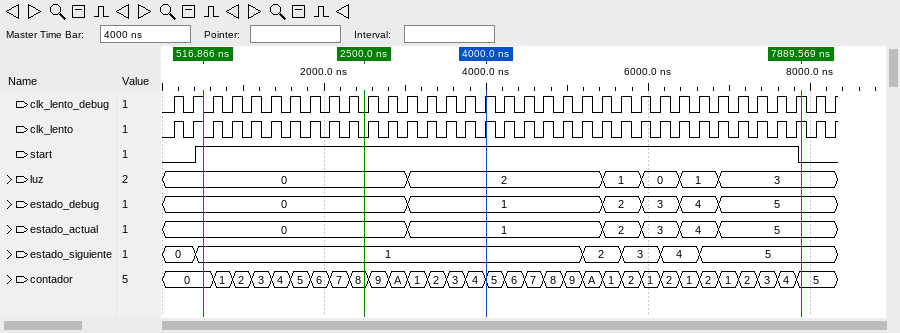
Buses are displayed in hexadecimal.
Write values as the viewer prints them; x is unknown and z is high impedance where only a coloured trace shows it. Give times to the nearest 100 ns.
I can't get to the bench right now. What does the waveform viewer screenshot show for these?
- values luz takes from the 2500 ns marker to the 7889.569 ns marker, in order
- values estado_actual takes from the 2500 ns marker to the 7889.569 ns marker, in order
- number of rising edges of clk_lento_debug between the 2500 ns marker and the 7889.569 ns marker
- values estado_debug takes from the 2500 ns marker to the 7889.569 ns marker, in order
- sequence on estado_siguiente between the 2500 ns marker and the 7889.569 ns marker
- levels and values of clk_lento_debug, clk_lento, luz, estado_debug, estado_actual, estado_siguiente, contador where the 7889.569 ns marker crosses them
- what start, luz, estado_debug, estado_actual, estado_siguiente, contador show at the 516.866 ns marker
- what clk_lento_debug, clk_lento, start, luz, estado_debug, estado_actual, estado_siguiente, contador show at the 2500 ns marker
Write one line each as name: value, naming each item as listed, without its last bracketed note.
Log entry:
values luz takes from the 2500 ns marker to the 7889.569 ns marker, in order: 0, 2, 1, 0, 1, 3
values estado_actual takes from the 2500 ns marker to the 7889.569 ns marker, in order: 0, 1, 2, 3, 4, 5
number of rising edges of clk_lento_debug between the 2500 ns marker and the 7889.569 ns marker: 23
values estado_debug takes from the 2500 ns marker to the 7889.569 ns marker, in order: 0, 1, 2, 3, 4, 5
sequence on estado_siguiente between the 2500 ns marker and the 7889.569 ns marker: 1, 2, 3, 4, 5
levels and values of clk_lento_debug, clk_lento, luz, estado_debug, estado_actual, estado_siguiente, contador where the 7889.569 ns marker crosses them: clk_lento_debug=1, clk_lento=1, luz=3, estado_debug=5, estado_actual=5, estado_siguiente=5, contador=5
what start, luz, estado_debug, estado_actual, estado_siguiente, contador show at the 516.866 ns marker: start=1, luz=0, estado_debug=0, estado_actual=0, estado_siguiente=1, contador=0
what clk_lento_debug, clk_lento, start, luz, estado_debug, estado_actual, estado_siguiente, contador show at the 2500 ns marker: clk_lento_debug=0, clk_lento=0, start=1, luz=0, estado_debug=0, estado_actual=0, estado_siguiente=1, contador=8
